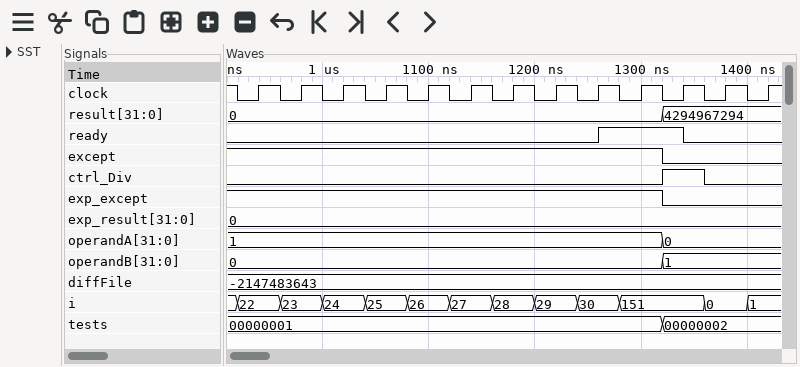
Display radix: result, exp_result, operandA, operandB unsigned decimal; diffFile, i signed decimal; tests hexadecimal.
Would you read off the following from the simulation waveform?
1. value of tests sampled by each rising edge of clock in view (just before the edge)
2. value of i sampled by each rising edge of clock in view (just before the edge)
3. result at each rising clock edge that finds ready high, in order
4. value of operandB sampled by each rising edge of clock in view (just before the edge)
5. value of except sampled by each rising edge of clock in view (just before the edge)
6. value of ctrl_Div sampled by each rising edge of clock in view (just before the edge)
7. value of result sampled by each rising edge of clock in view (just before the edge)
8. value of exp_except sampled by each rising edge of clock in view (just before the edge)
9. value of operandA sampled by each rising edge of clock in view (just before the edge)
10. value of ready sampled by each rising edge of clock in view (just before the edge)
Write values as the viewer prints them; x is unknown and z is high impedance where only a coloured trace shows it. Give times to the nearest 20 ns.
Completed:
00000001, 00000001, 00000001, 00000001, 00000001, 00000001, 00000001, 00000001, 00000001, 00000001, 00000002, 00000002, 00000002
22, 23, 24, 25, 26, 27, 28, 29, 30, 151, 151, 0, 1
0, 4294967294
0, 0, 0, 0, 0, 0, 0, 0, 0, 0, 1, 1, 1
1 1 1 1 1 1 1 1 1 1 0 0 0
0 0 0 0 0 0 0 0 0 0 1 0 0
0, 0, 0, 0, 0, 0, 0, 0, 0, 0, 4294967294, 4294967294, 4294967294
1 1 1 1 1 1 1 1 1 1 0 0 0
1, 1, 1, 1, 1, 1, 1, 1, 1, 1, 0, 0, 0
0 0 0 0 0 0 0 0 0 1 1 0 0
